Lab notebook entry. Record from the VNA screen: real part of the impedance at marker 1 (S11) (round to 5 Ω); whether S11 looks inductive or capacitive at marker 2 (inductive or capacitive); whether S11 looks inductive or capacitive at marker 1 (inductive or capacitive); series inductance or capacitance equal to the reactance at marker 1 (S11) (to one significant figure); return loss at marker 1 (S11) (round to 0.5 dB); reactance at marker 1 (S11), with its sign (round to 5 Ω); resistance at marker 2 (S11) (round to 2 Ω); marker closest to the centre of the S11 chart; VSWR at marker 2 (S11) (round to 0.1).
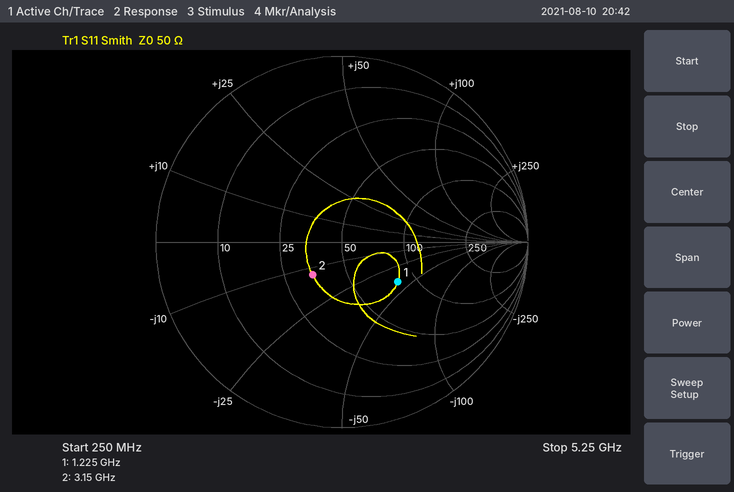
80 Ω
capacitive
capacitive
3 pF
8.5 dB
-40 Ω
34 Ω
marker 2
1.6
